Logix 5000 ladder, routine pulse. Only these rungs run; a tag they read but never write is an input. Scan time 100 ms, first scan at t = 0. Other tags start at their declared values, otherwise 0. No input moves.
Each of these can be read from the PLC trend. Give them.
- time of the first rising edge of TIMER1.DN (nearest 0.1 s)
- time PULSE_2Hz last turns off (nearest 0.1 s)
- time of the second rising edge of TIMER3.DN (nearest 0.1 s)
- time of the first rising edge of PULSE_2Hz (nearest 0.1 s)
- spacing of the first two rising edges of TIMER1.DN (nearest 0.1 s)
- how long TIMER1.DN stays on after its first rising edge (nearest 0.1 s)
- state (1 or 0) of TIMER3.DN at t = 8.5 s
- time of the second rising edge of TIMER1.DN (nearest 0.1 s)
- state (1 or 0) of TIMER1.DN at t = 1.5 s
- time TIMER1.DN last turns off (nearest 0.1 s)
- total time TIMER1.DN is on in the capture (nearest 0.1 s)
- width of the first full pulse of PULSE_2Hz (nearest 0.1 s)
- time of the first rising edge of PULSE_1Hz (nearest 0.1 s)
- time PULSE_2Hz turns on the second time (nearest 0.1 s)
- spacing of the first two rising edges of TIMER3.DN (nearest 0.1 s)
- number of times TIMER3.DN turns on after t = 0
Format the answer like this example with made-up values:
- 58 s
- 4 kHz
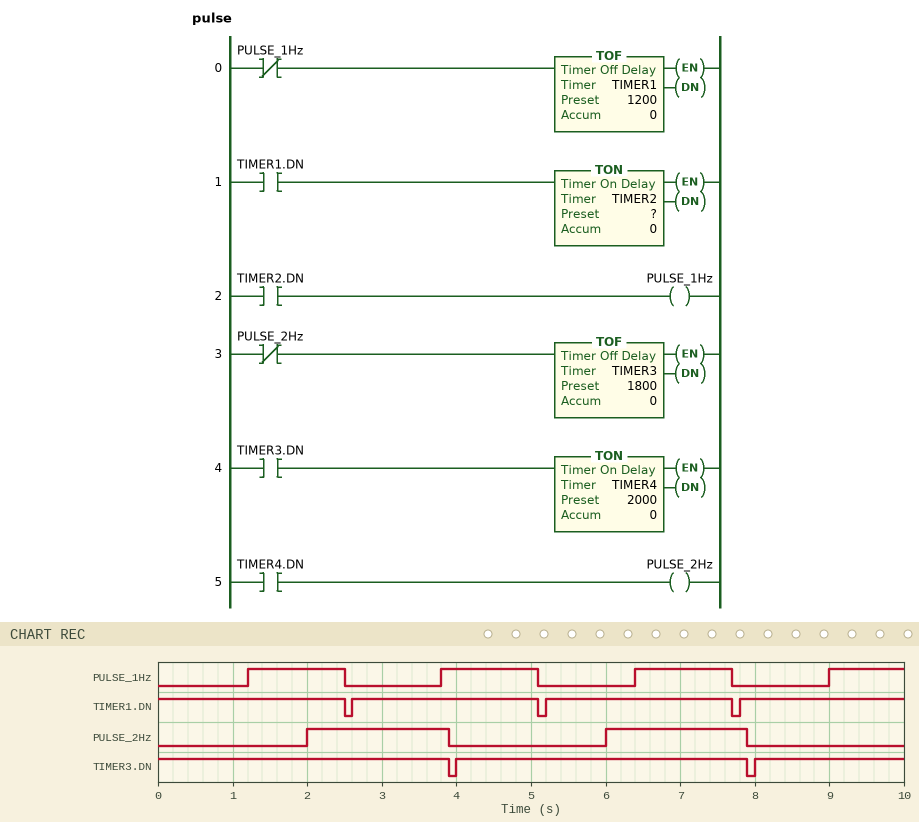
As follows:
- 2.6 s
- 7.9 s
- 8.0 s
- 2.0 s
- 2.6 s
- 2.5 s
- 1
- 5.2 s
- 1
- 7.7 s
- 9.7 s
- 1.9 s
- 1.2 s
- 6.0 s
- 4.0 s
- 2
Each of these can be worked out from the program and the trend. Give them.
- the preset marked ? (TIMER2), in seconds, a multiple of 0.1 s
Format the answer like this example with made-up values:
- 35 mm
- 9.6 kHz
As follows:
- 1.2 s
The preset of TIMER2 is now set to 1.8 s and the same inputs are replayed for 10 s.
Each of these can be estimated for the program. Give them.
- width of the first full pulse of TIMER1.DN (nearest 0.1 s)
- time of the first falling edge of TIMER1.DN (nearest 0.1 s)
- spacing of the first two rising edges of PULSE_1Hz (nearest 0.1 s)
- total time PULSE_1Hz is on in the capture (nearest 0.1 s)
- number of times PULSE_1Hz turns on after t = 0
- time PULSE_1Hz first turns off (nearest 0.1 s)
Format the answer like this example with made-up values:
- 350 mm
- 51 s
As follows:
- 3.1 s
- 3.1 s
- 3.2 s
- 3.9 s
- 3
- 3.1 s
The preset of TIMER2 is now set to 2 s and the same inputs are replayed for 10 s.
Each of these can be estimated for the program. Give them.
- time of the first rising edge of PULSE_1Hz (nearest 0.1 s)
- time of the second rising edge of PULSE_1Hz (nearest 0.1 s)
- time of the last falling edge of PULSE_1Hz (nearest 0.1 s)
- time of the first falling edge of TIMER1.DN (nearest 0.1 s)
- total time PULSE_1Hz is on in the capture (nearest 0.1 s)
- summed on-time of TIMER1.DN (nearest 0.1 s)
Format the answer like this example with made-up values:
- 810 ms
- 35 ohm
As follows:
- 2.0 s
- 5.4 s
- 6.7 s
- 3.3 s
- 3.8 s
- 9.8 s
